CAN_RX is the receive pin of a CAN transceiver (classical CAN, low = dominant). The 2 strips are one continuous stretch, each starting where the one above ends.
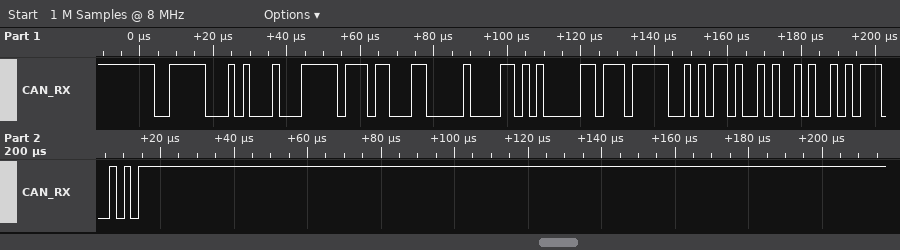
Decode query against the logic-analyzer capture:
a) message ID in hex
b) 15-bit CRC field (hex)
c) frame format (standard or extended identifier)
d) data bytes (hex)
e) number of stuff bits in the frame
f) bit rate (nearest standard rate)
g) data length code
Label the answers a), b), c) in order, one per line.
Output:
a) 0x3E5
b) 0x2572
c) standard
d) FF 63 00 6A 0B BE AD 29
e) 5
f) 500 kbit/s
g) 8
